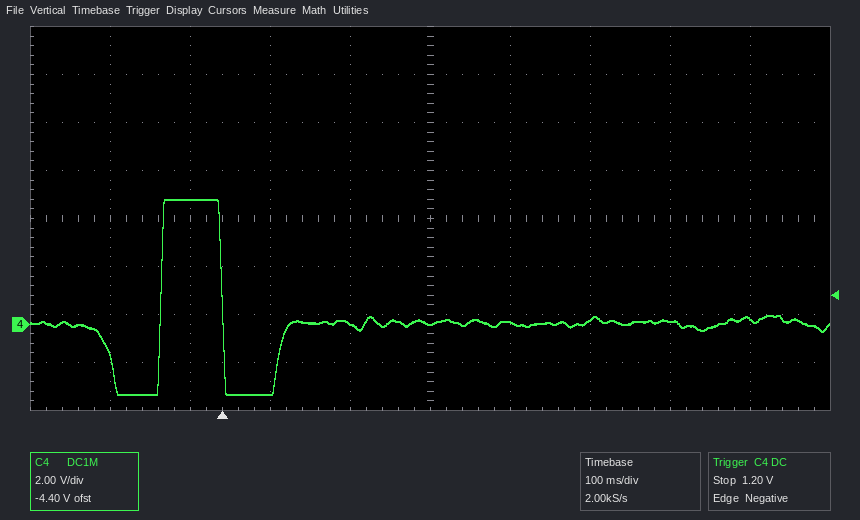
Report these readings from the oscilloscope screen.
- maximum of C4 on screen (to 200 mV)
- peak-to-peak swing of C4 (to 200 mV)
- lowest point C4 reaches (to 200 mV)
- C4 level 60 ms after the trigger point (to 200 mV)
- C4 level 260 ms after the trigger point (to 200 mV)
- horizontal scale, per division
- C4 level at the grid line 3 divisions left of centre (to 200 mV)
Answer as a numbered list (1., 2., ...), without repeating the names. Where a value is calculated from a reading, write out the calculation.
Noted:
1. 5.2 V
2. 5.2 V − (-3.0 V) = 8.2 V
3. -3.0 V
4. -2.8 V
5. 0.0 V
6. 100 ms
7. 5.2 V
